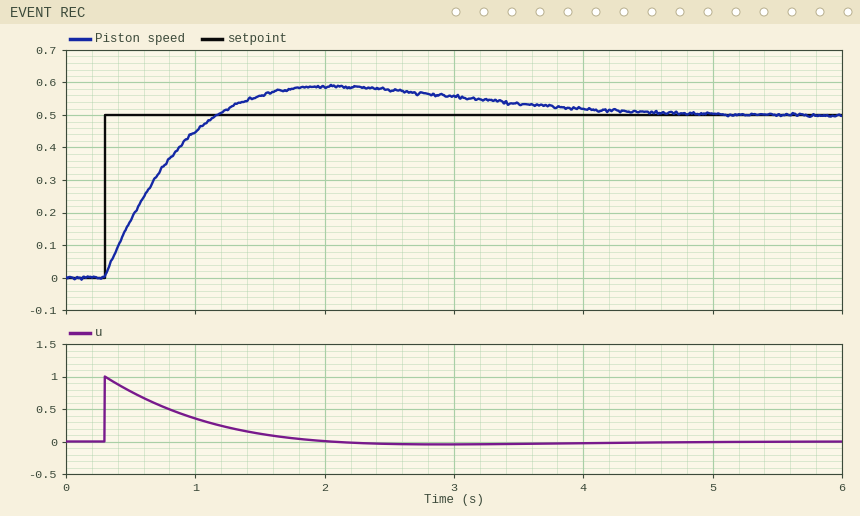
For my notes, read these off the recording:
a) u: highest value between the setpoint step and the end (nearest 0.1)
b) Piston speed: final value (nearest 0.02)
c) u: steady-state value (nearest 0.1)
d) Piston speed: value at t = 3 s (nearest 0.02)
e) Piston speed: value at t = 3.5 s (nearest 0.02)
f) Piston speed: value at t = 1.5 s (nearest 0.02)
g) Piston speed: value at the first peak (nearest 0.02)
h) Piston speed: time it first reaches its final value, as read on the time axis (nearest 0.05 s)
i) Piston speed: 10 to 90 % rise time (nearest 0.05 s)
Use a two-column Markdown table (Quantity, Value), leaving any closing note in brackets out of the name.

| Quantity | Value |
|---|---|
| u: highest value between the setpoint step and the end | 1.0 |
| Piston speed: final value | 0.50 |
| u: steady-state value | 0.0 |
| Piston speed: value at t = 3 s | 0.56 |
| Piston speed: value at t = 3.5 s | 0.54 |
| Piston speed: value at t = 1.5 s | 0.56 |
| Piston speed: value at the first peak | 0.58 |
| Piston speed: time it first reaches its final value, as read on the time axis | 1.15 s |
| Piston speed: 10 to 90 % rise time | 0.65 s |
